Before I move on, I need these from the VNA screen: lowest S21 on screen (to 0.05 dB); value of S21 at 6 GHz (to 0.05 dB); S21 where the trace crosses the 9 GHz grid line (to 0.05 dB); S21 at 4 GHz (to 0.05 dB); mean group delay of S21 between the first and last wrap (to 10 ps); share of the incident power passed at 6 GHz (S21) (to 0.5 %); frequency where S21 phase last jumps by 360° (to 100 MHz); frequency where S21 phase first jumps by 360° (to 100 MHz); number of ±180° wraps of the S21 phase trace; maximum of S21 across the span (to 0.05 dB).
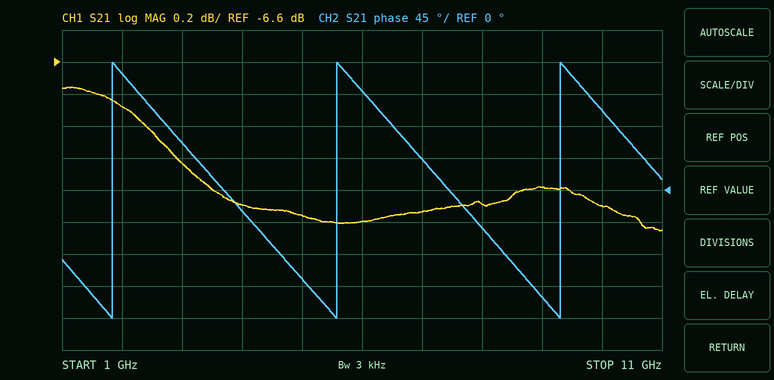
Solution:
-7.65 dB
-7.60 dB
-7.40 dB
-7.50 dB
270 ps
17.5 %
9.3 GHz
1.8 GHz
3
-6.75 dB
